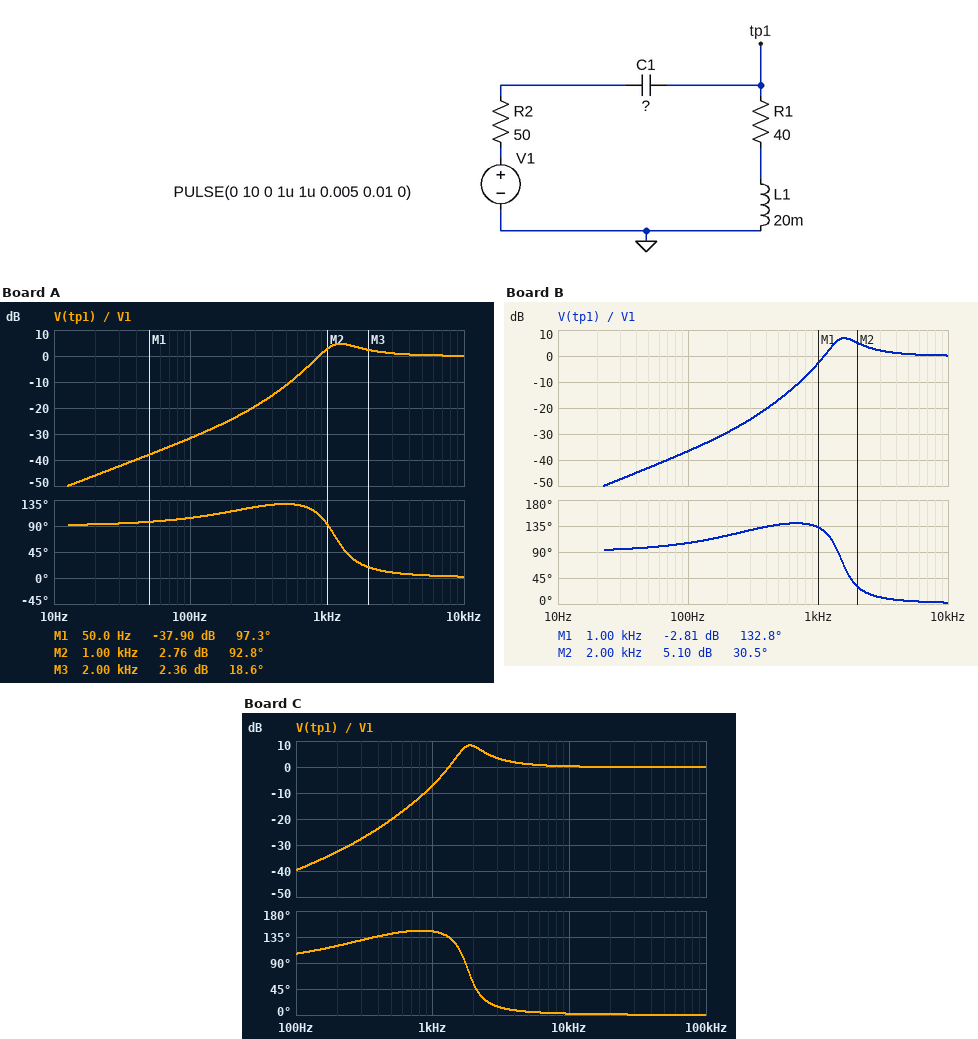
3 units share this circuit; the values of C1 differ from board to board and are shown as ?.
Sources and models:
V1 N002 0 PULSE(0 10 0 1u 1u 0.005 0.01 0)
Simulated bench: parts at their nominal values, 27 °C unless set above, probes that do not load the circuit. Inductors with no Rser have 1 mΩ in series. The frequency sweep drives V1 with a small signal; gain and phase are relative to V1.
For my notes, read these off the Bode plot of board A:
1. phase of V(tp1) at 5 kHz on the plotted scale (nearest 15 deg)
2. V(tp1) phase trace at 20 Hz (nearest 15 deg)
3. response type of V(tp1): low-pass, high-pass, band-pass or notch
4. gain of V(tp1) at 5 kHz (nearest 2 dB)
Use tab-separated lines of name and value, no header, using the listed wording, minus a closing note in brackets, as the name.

phase of V(tp1) at 5 kHz on the plotted scale	0 deg
V(tp1) phase trace at 20 Hz	90 deg
response type of V(tp1): low-pass, high-pass, band-pass or notch	high-pass
gain of V(tp1) at 5 kHz	0 dB
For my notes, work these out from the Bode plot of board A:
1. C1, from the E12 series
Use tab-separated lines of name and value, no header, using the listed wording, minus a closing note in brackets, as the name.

C1, from the E12 series	1 µF
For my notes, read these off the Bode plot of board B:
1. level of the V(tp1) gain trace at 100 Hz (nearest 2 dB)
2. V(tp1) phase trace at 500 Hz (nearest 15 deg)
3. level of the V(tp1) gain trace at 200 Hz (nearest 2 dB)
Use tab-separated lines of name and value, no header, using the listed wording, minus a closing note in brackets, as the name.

level of the V(tp1) gain trace at 100 Hz	-36 dB
V(tp1) phase trace at 500 Hz	135 deg
level of the V(tp1) gain trace at 200 Hz	-30 dB
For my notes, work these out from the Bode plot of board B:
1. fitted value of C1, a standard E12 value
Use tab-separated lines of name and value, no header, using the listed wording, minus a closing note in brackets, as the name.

fitted value of C1, a standard E12 value	560 nF
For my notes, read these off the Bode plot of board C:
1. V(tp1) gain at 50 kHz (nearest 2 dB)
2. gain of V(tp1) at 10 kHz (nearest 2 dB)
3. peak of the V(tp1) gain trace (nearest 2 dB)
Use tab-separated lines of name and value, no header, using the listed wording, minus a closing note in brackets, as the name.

V(tp1) gain at 50 kHz	0 dB
gain of V(tp1) at 10 kHz	0 dB
peak of the V(tp1) gain trace	8 dB
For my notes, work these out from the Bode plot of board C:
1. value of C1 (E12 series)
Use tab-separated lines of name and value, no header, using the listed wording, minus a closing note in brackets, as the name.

value of C1	390 nF
